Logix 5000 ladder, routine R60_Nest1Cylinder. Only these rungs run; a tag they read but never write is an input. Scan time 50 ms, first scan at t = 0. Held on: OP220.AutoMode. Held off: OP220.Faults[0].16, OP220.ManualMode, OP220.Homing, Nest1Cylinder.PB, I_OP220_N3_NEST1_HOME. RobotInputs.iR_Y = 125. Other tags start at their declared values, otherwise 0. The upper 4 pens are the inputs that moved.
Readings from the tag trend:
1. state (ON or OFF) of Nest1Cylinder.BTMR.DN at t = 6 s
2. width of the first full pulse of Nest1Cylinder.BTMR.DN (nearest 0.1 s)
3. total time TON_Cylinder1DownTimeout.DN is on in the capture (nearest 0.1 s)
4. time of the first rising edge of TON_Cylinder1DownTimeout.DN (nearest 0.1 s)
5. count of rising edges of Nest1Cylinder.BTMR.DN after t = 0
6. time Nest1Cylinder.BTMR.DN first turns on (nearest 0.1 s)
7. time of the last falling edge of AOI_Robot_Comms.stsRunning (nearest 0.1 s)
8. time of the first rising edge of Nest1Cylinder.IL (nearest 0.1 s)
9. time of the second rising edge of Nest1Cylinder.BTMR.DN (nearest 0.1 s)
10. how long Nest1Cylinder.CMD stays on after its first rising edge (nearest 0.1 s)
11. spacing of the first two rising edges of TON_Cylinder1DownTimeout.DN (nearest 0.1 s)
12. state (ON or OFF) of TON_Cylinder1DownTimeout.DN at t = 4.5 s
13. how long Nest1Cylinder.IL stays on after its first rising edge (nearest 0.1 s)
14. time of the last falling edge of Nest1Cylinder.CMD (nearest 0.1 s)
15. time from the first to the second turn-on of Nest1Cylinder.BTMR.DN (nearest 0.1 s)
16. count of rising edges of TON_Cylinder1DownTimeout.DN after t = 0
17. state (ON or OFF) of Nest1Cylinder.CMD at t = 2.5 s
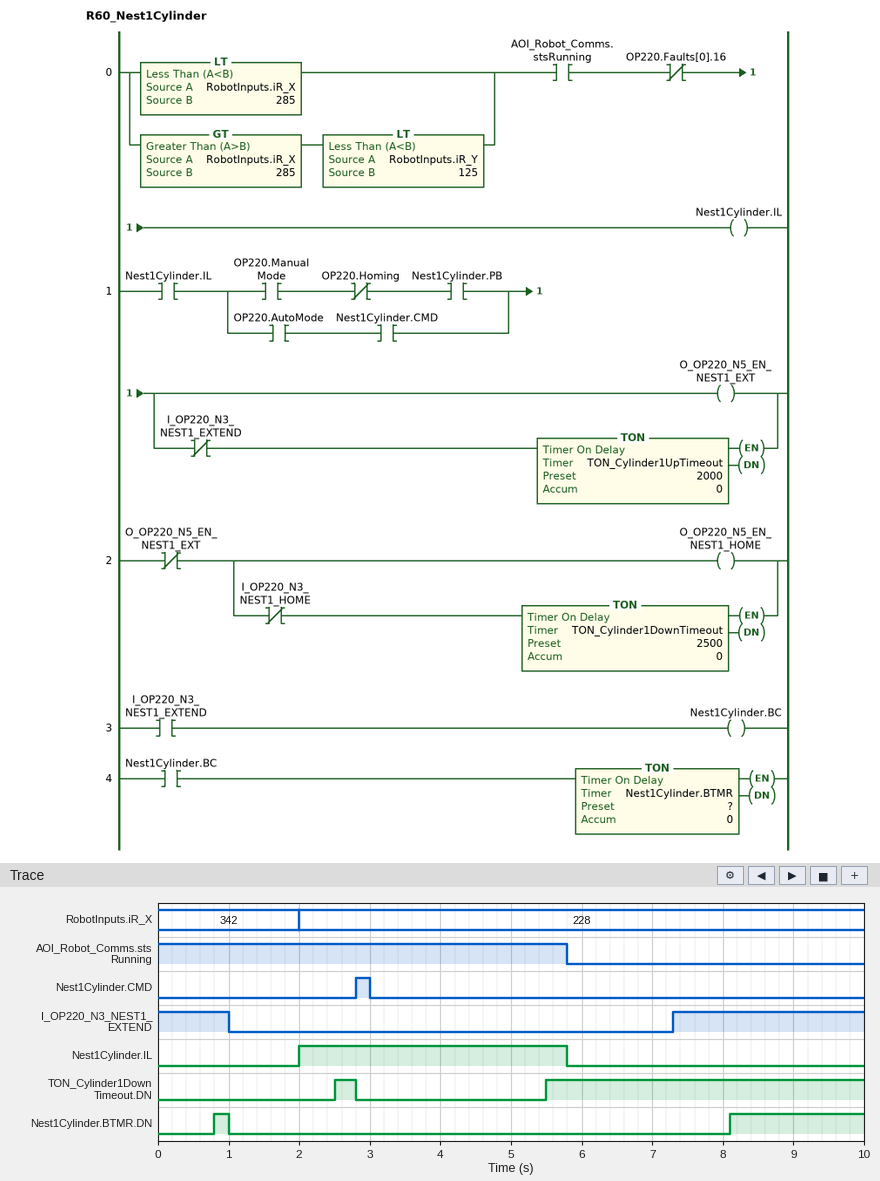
OFF
0.2 s
4.8 s
2.5 s
2
0.8 s
5.8 s
2.0 s
8.1 s
0.2 s
3.0 s
OFF
3.8 s
3.0 s
7.3 s
2
OFF
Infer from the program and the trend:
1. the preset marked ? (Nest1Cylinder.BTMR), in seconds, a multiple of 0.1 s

0.8 s
